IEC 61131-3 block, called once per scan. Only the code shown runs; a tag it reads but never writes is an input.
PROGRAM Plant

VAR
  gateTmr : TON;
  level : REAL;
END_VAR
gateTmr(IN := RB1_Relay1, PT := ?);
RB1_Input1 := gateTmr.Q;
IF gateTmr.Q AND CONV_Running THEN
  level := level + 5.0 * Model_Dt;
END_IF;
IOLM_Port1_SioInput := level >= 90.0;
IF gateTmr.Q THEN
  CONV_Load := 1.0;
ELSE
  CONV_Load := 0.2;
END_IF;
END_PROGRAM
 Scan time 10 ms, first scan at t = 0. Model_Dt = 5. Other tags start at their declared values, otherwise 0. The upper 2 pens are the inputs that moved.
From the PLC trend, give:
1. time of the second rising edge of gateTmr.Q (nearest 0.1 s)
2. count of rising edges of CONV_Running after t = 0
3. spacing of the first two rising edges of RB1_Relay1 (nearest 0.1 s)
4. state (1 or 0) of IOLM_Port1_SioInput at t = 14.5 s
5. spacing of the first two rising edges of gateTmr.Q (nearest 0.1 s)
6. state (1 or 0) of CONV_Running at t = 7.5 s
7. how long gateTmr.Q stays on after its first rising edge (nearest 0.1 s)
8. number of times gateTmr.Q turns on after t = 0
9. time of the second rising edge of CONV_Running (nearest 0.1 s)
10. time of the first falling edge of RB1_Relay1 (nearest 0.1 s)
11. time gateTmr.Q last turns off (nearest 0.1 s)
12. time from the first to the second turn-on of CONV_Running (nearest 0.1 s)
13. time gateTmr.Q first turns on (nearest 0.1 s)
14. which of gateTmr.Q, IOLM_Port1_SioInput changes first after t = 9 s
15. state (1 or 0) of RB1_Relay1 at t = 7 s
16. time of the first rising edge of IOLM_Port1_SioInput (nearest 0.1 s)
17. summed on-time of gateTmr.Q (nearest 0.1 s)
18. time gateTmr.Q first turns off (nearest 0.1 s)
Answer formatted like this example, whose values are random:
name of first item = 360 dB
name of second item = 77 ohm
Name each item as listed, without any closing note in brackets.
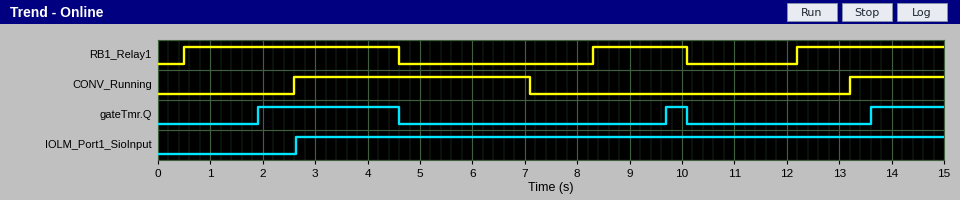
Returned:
time of the second rising edge of gateTmr.Q = 9.7 s
count of rising edges of CONV_Running after t = 0 = 2
spacing of the first two rising edges of RB1_Relay1 = 7.8 s
state (1 or 0) of IOLM_Port1_SioInput at t = 14.5 s = 1
spacing of the first two rising edges of gateTmr.Q = 7.8 s
state (1 or 0) of CONV_Running at t = 7.5 s = 0
how long gateTmr.Q stays on after its first rising edge = 2.7 s
number of times gateTmr.Q turns on after t = 0 = 3
time of the second rising edge of CONV_Running = 13.2 s
time of the first falling edge of RB1_Relay1 = 4.6 s
time gateTmr.Q last turns off = 10.1 s
time from the first to the second turn-on of CONV_Running = 10.6 s
time gateTmr.Q first turns on = 1.9 s
which of gateTmr.Q, IOLM_Port1_SioInput changes first after t = 9 s = gateTmr.Q
state (1 or 0) of RB1_Relay1 at t = 7 s = 0
time of the first rising edge of IOLM_Port1_SioInput = 2.6 s
summed on-time of gateTmr.Q = 4.5 s
time gateTmr.Q first turns off = 4.6 s
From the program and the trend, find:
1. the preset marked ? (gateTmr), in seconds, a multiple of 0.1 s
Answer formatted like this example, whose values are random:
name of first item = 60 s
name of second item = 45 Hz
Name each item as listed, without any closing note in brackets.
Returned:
the preset marked ? (gateTmr), in seconds, a multiple of 0.1 s = 1.4 s
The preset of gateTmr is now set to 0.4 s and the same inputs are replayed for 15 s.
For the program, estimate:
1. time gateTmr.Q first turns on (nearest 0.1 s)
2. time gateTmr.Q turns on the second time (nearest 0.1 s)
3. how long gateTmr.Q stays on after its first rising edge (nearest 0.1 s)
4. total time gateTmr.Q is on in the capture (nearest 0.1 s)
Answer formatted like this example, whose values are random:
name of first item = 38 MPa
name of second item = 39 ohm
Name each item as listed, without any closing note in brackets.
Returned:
time gateTmr.Q first turns on = 0.9 s
time gateTmr.Q turns on the second time = 8.7 s
how long gateTmr.Q stays on after its first rising edge = 3.7 s
total time gateTmr.Q is on in the capture = 7.5 s
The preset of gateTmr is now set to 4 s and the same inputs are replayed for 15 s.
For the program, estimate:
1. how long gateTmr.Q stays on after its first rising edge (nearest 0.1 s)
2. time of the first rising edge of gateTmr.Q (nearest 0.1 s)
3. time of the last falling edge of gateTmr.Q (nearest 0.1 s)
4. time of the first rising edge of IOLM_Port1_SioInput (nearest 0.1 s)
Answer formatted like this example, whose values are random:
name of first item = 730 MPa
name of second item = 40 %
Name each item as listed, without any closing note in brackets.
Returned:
how long gateTmr.Q stays on after its first rising edge = 0.1 s
time of the first rising edge of gateTmr.Q = 4.5 s
time of the last falling edge of gateTmr.Q = 4.6 s
time of the first rising edge of IOLM_Port1_SioInput = 4.5 s
